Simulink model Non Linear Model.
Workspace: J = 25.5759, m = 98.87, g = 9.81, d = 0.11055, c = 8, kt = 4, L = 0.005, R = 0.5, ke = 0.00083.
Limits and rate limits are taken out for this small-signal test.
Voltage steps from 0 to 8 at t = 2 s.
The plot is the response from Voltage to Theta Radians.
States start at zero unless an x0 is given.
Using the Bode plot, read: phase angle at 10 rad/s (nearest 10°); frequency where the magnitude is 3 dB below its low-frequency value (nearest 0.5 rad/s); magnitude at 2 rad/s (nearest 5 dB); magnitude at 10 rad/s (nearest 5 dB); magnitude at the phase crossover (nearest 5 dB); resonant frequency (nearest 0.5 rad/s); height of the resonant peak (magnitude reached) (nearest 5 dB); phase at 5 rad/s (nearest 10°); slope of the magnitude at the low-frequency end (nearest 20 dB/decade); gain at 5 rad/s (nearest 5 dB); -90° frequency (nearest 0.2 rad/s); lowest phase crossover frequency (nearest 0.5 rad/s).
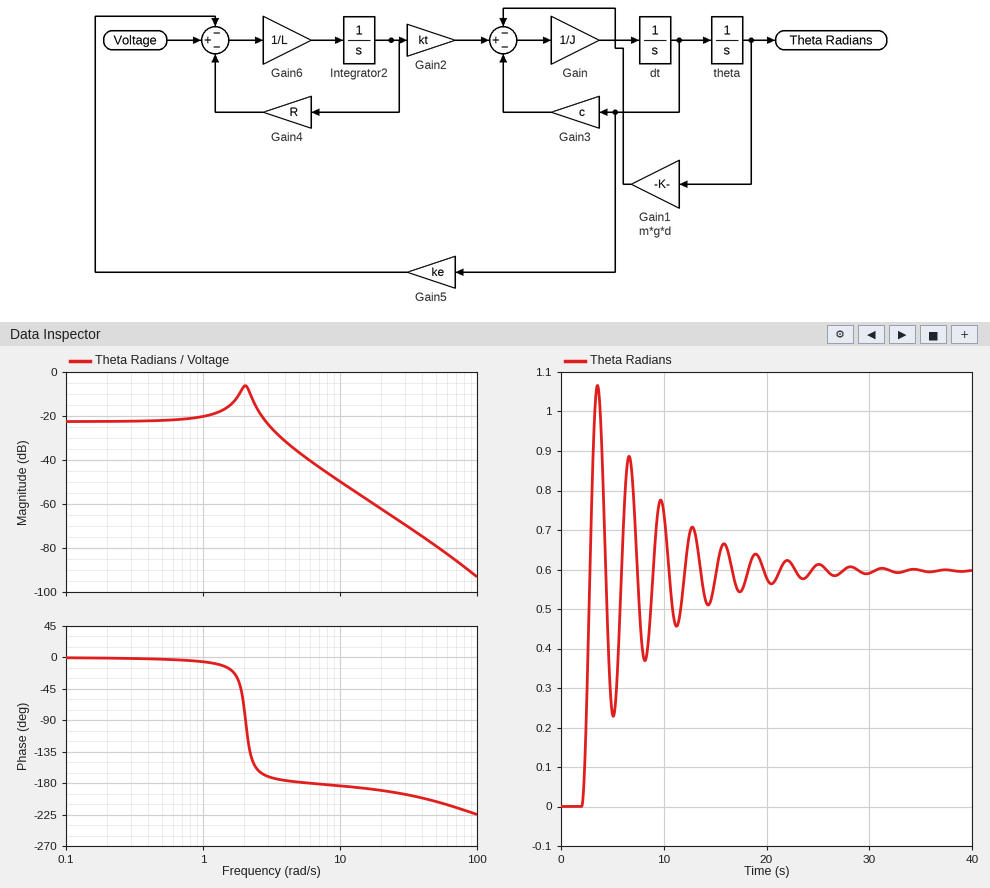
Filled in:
-180°
3.0 rad/s
-5 dB
-50 dB
-40 dB
2.0 rad/s
-5 dB
-180°
0 dB/decade
-35 dB
2.0 rad/s
6.0 rad/s
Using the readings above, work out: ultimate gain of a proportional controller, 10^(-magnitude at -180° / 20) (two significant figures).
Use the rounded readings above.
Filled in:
100
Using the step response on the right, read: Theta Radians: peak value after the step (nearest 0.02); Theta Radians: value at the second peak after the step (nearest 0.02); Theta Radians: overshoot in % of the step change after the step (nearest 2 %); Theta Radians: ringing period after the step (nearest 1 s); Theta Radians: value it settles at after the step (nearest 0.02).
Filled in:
1.06
0.88
78 %
3 s
0.60
